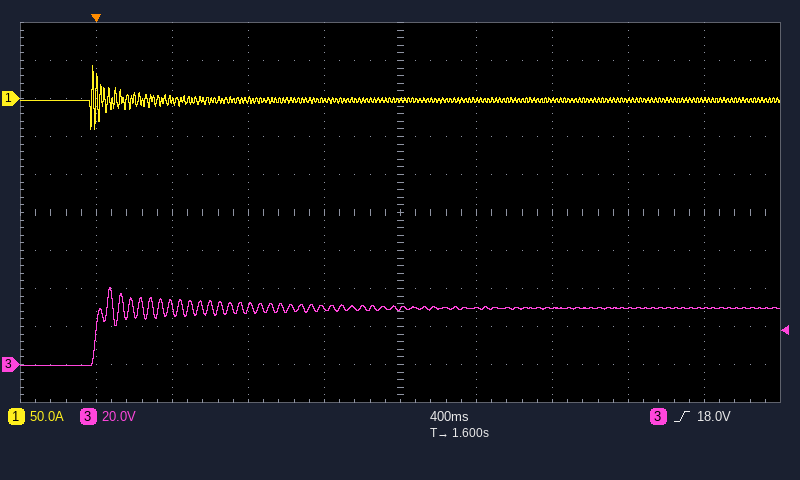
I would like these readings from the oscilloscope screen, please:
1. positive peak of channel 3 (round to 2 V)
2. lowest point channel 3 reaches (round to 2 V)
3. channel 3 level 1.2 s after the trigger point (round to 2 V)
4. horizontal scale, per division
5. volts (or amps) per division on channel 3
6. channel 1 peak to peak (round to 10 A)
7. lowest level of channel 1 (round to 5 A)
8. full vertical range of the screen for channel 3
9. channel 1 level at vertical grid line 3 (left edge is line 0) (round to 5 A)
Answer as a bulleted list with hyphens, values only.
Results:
- 40 V
- 0 V
- 30 V
- 400 ms
- 20 V
- 80 A
- -40 A
- 200 V
- 0 A
